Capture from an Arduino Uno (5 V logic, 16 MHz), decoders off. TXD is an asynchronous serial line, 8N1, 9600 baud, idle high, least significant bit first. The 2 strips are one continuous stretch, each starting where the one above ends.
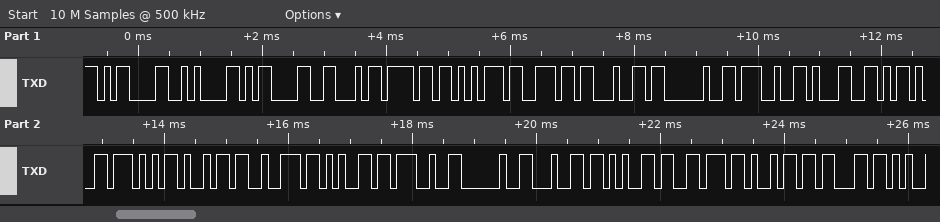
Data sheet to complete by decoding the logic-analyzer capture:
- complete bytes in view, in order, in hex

0x0D 0x0A 0x0D 0x46 0x6F 0x75 0x6E 0x64 0x20 0x27 0x31 0x2D 0x57 0x69 0x72 0x65 0x27 0x20 0x64 0x65 0x76 0x69 0x63
